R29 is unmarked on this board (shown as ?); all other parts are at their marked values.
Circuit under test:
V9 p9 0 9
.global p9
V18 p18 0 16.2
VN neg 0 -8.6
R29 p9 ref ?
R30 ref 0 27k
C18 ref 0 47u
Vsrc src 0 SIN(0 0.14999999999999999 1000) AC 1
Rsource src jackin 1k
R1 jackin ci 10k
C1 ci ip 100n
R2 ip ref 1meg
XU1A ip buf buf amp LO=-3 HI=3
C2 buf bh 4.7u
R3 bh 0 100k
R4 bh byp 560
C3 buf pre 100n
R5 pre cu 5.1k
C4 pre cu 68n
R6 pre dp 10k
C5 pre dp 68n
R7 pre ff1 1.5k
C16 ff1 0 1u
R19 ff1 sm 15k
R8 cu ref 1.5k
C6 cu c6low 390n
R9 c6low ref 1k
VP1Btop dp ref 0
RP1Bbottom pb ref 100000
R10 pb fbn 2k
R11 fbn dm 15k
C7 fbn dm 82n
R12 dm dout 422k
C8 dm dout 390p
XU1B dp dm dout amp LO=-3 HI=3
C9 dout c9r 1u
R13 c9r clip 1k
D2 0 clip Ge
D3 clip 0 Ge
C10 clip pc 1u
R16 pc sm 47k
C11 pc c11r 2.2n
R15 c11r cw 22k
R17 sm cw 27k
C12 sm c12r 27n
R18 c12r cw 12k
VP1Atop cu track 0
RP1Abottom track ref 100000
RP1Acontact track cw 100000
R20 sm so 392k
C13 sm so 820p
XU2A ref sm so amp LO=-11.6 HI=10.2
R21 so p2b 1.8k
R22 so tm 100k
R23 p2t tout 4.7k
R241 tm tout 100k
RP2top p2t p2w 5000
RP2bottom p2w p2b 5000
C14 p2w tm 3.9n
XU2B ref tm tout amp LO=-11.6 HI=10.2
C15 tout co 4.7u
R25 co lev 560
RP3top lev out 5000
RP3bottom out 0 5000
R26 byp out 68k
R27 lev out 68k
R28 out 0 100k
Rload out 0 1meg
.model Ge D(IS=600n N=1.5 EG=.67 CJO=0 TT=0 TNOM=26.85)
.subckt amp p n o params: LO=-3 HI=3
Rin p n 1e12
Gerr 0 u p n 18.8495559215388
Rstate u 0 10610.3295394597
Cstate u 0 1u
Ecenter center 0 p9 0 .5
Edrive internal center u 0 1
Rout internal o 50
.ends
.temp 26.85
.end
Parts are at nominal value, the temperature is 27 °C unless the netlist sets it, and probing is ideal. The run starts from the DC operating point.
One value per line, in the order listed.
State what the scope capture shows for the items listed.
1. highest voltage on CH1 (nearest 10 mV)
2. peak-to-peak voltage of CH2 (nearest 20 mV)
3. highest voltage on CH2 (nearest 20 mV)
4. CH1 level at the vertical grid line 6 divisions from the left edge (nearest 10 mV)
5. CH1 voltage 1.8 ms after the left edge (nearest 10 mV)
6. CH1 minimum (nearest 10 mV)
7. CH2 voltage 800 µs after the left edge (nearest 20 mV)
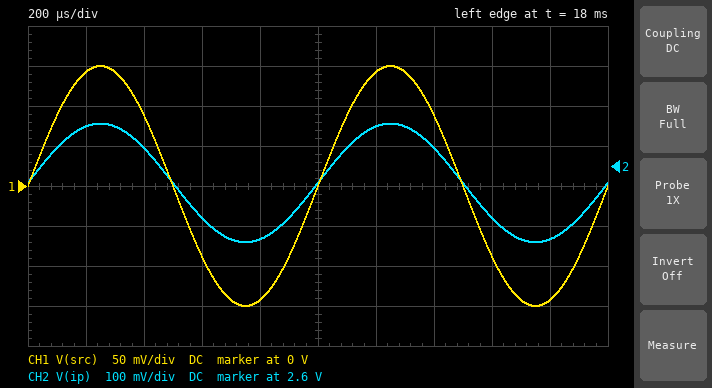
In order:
150 mV
300 mV
2.70 V
140 mV
-140 mV
-150 mV
2.42 V
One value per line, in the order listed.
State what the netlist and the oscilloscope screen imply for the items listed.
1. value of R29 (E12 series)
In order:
68 kΩ
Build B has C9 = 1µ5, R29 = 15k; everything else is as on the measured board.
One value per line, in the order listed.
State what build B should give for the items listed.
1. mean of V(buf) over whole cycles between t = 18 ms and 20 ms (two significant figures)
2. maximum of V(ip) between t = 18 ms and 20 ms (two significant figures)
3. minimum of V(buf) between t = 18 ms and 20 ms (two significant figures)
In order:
5.8 V
5.9 V
5.6 V
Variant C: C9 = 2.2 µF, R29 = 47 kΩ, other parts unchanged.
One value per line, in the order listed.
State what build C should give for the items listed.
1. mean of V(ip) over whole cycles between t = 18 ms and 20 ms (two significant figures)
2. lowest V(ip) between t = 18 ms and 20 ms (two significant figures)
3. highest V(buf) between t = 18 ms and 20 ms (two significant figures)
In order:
3.3 V
3.1 V
3.4 V
